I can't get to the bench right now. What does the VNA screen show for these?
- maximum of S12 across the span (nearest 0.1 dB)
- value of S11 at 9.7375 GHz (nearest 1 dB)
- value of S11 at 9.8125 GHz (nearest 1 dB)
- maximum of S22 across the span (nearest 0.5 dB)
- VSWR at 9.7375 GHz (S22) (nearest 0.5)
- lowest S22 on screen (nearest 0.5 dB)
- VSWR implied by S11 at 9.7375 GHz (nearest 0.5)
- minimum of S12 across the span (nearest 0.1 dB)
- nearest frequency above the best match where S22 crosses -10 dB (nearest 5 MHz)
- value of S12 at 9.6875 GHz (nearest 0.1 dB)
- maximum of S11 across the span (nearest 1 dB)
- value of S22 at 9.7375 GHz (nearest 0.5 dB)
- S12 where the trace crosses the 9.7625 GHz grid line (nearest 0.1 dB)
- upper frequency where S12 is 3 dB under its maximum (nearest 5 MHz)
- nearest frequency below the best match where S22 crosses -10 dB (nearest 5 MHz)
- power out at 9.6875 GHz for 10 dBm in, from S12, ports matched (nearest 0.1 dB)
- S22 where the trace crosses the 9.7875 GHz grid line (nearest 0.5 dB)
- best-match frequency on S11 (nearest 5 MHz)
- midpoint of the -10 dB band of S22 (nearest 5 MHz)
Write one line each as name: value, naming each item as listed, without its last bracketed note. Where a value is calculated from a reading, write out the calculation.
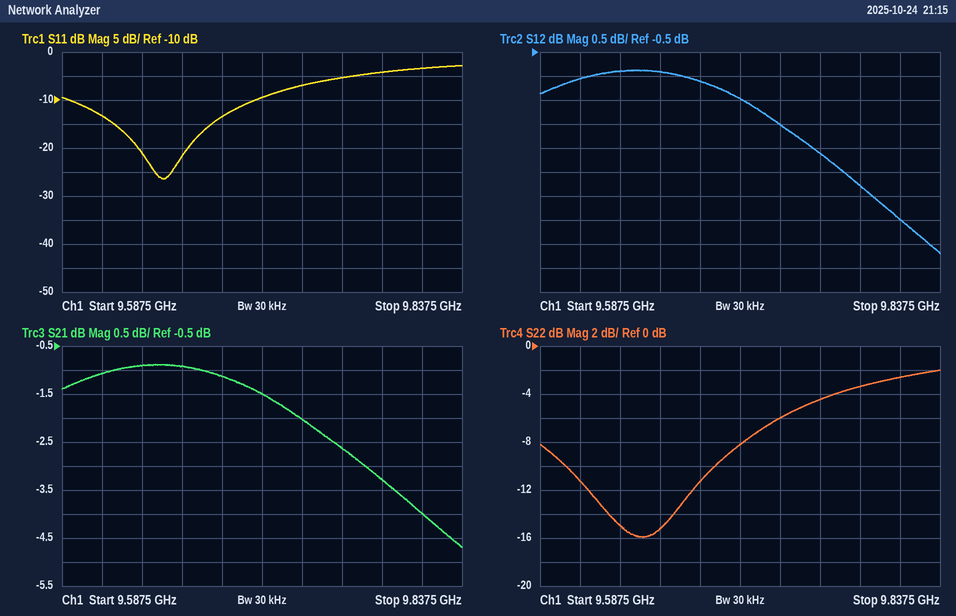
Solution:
maximum of S12 across the span: -0.9 dB
value of S11 at 9.7375 GHz: -7 dB
value of S11 at 9.8125 GHz: -3 dB
maximum of S22 across the span: -2.0 dB
VSWR at 9.7375 GHz (S22): |Γ| = 10^(-6/20) = 0.5012; VSWR = (1 + 0.5012)/(1 − 0.5012) ≈ 3.0
lowest S22 on screen: -16.0 dB
VSWR implied by S11 at 9.7375 GHz: |Γ| = 10^(-7/20) = 0.4467; VSWR = (1 + 0.4467)/(1 − 0.4467) ≈ 2.61, so 2.5 to the nearest 0.5
minimum of S12 across the span: -4.7 dB
nearest frequency above the best match where S22 crosses -10 dB: 9.695 GHz
value of S12 at 9.6875 GHz: -1.1 dB
maximum of S11 across the span: -3 dB
value of S22 at 9.7375 GHz: -6.0 dB
S12 where the trace crosses the 9.7625 GHz grid line: -2.6 dB
upper frequency where S12 is 3 dB under its maximum: 9.810 GHz
nearest frequency below the best match where S22 crosses -10 dB: 9.605 GHz
power out at 9.6875 GHz for 10 dBm in, from S12, ports matched: 10 dBm + (-1.1 dB) = 8.9 dBm
S22 where the trace crosses the 9.7875 GHz grid line: -3.5 dB
best-match frequency on S11: 9.650 GHz
midpoint of the -10 dB band of S22: 9.650 GHz
